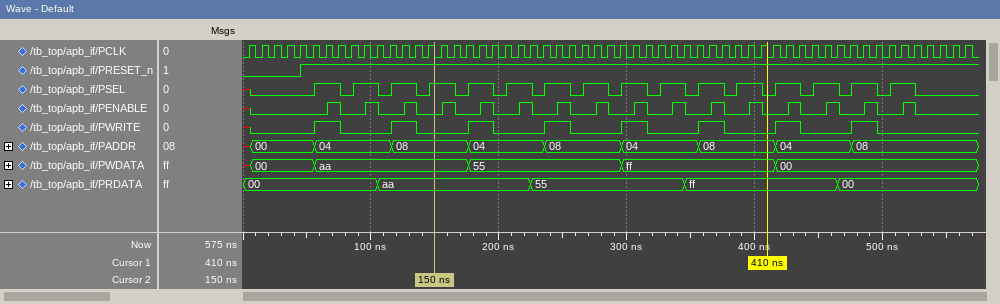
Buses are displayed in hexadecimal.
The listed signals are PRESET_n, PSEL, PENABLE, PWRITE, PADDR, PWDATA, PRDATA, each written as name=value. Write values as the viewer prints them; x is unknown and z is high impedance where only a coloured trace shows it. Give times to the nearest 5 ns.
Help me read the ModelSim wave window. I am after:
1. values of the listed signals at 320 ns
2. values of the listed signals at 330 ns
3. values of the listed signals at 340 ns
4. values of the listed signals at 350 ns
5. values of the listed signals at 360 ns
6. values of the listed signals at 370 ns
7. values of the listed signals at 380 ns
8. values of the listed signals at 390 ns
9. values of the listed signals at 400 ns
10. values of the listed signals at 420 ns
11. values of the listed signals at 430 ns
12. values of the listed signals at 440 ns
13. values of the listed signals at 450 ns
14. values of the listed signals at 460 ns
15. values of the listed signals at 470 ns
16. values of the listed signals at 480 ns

PRESET_n=1, PSEL=0, PENABLE=0, PWRITE=0, PADDR=04, PWDATA=ff, PRDATA=55
PRESET_n=1, PSEL=1, PENABLE=0, PWRITE=0, PADDR=04, PWDATA=ff, PRDATA=55
PRESET_n=1, PSEL=1, PENABLE=1, PWRITE=0, PADDR=04, PWDATA=ff, PRDATA=55
PRESET_n=1, PSEL=0, PENABLE=0, PWRITE=0, PADDR=04, PWDATA=ff, PRDATA=ff
PRESET_n=1, PSEL=1, PENABLE=0, PWRITE=1, PADDR=08, PWDATA=ff, PRDATA=ff
PRESET_n=1, PSEL=1, PENABLE=1, PWRITE=1, PADDR=08, PWDATA=ff, PRDATA=ff
PRESET_n=1, PSEL=0, PENABLE=0, PWRITE=0, PADDR=08, PWDATA=ff, PRDATA=ff
PRESET_n=1, PSEL=1, PENABLE=0, PWRITE=0, PADDR=08, PWDATA=ff, PRDATA=ff
PRESET_n=1, PSEL=1, PENABLE=1, PWRITE=0, PADDR=08, PWDATA=ff, PRDATA=ff
PRESET_n=1, PSEL=1, PENABLE=0, PWRITE=1, PADDR=04, PWDATA=00, PRDATA=ff
PRESET_n=1, PSEL=1, PENABLE=1, PWRITE=1, PADDR=04, PWDATA=00, PRDATA=ff
PRESET_n=1, PSEL=0, PENABLE=0, PWRITE=0, PADDR=04, PWDATA=00, PRDATA=ff
PRESET_n=1, PSEL=1, PENABLE=0, PWRITE=0, PADDR=04, PWDATA=00, PRDATA=ff
PRESET_n=1, PSEL=1, PENABLE=1, PWRITE=0, PADDR=04, PWDATA=00, PRDATA=ff
PRESET_n=1, PSEL=0, PENABLE=0, PWRITE=0, PADDR=04, PWDATA=00, PRDATA=00
PRESET_n=1, PSEL=1, PENABLE=0, PWRITE=1, PADDR=08, PWDATA=00, PRDATA=00
